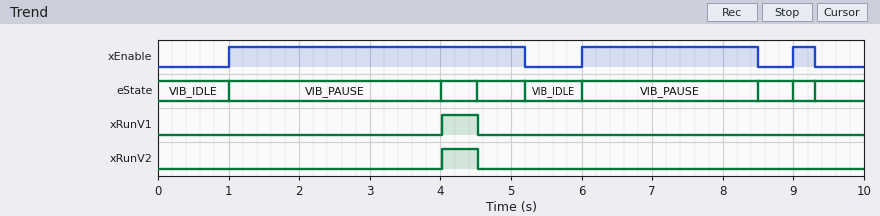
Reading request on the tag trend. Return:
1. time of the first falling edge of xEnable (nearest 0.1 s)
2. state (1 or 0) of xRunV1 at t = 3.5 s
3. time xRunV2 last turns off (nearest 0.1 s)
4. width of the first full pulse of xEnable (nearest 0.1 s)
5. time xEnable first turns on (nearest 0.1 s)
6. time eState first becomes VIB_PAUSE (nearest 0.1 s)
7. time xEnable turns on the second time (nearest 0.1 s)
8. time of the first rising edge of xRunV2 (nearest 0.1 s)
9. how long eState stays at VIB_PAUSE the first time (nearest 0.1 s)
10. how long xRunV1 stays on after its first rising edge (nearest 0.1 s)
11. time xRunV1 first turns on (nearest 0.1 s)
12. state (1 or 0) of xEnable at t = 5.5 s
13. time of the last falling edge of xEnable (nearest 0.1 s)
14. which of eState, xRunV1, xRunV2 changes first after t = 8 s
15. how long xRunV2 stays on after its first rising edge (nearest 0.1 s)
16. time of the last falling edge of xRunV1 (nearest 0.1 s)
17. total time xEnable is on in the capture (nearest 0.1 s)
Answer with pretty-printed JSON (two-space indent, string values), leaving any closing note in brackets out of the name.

{
  "time of the first falling edge of xEnable": "5.2 s",
  "state (1 or 0) of xRunV1 at t = 3.5 s": "0",
  "time xRunV2 last turns off": "4.5 s",
  "width of the first full pulse of xEnable": "4.2 s",
  "time xEnable first turns on": "1.0 s",
  "time eState first becomes VIB_PAUSE": "1.0 s",
  "time xEnable turns on the second time": "6.0 s",
  "time of the first rising edge of xRunV2": "4.0 s",
  "how long eState stays at VIB_PAUSE the first time": "3.0 s",
  "how long xRunV1 stays on after its first rising edge": "0.5 s",
  "time xRunV1 first turns on": "4.0 s",
  "state (1 or 0) of xEnable at t = 5.5 s": "0",
  "time of the last falling edge of xEnable": "9.3 s",
  "which of eState, xRunV1, xRunV2 changes first after t = 8 s": "eState",
  "how long xRunV2 stays on after its first rising edge": "0.5 s",
  "time of the last falling edge of xRunV1": "4.5 s",
  "total time xEnable is on in the capture": "7.0 s"
}
